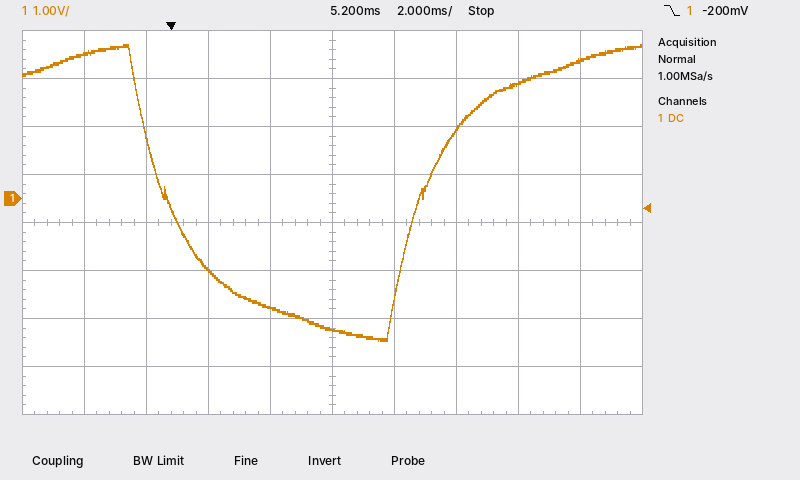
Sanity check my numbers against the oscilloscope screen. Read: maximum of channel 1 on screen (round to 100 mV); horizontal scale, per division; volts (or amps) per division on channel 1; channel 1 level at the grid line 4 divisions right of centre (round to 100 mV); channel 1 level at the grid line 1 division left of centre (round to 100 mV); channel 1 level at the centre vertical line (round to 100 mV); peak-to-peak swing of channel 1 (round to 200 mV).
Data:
3.2 V
2 ms
1 V
2.9 V
-2.3 V
-2.7 V
6.2 V
